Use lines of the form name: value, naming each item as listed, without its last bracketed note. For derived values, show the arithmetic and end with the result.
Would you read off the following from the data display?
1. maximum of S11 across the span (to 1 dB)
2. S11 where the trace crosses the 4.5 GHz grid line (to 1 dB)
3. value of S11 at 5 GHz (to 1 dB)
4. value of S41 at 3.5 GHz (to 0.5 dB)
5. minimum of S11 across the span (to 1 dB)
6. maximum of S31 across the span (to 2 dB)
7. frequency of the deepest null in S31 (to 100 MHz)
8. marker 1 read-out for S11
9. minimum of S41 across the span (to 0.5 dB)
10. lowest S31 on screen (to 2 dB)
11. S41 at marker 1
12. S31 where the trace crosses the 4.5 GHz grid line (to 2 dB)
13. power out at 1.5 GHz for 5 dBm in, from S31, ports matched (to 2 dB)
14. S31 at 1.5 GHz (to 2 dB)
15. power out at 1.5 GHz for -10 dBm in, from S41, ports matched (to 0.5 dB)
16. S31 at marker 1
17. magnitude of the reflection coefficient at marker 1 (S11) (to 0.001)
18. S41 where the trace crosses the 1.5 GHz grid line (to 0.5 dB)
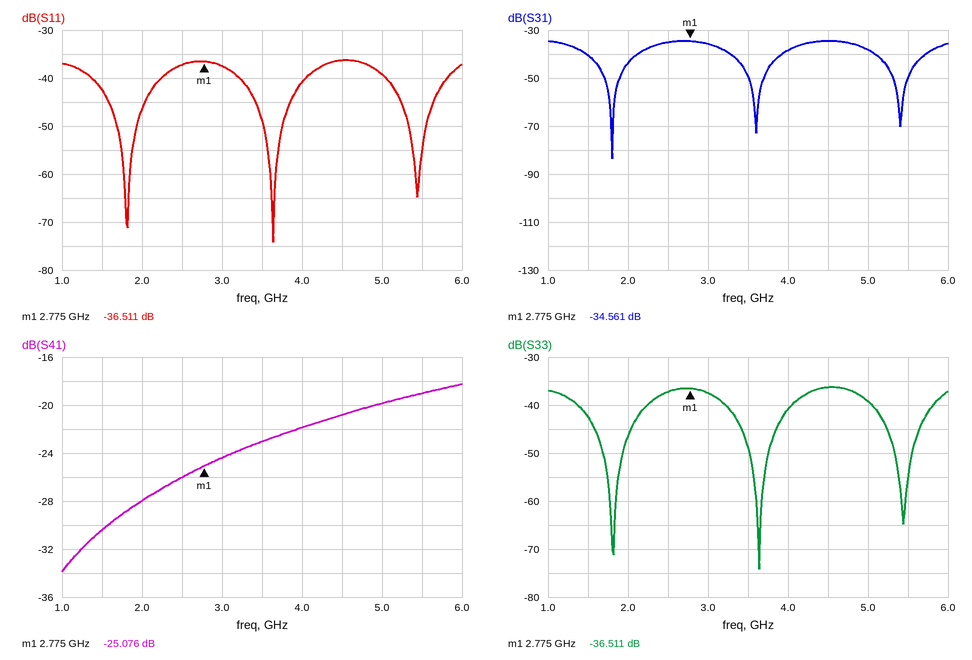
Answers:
maximum of S11 across the span: -36 dB
S11 where the trace crosses the 4.5 GHz grid line: -36 dB
value of S11 at 5 GHz: -39 dB
value of S41 at 3.5 GHz: -23.0 dB
minimum of S11 across the span: -74 dB
maximum of S31 across the span: -34 dB
frequency of the deepest null in S31: 1.8 GHz
marker 1 read-out for S11: -36.511 dB
minimum of S41 across the span: -34.0 dB
lowest S31 on screen: -84 dB
S41 at marker 1: -25.076 dB
S31 where the trace crosses the 4.5 GHz grid line: -34 dB
power out at 1.5 GHz for 5 dBm in, from S31, ports matched: 5 dBm + (-40 dB) = -36 dBm
S31 at 1.5 GHz: -40 dB
power out at 1.5 GHz for -10 dBm in, from S41, ports matched: -10 dBm + (-30.5 dB) = -40.5 dBm
S31 at marker 1: -34.561 dB
magnitude of the reflection coefficient at marker 1 (S11): 10^(-36.511/20) ≈ 0.015
S41 where the trace crosses the 1.5 GHz grid line: -30.5 dB
